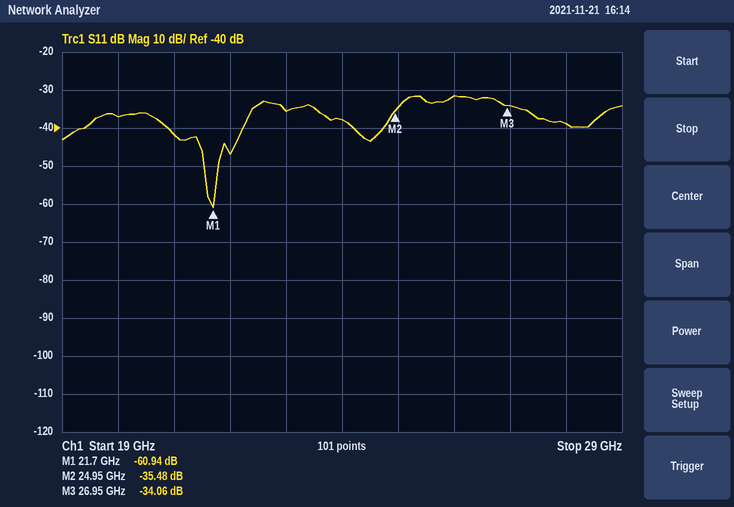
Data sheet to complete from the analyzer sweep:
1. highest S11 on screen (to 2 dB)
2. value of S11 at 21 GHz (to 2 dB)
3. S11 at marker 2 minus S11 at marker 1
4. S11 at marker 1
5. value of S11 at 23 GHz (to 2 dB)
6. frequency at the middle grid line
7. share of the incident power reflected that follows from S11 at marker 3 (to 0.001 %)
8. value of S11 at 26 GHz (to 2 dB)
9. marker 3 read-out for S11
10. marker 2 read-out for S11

-32 dB
-42 dB
25.46 dB
-60.94 dB
-36 dB
24 GHz
0.039 %
-32 dB
-34.06 dB
-35.48 dB
